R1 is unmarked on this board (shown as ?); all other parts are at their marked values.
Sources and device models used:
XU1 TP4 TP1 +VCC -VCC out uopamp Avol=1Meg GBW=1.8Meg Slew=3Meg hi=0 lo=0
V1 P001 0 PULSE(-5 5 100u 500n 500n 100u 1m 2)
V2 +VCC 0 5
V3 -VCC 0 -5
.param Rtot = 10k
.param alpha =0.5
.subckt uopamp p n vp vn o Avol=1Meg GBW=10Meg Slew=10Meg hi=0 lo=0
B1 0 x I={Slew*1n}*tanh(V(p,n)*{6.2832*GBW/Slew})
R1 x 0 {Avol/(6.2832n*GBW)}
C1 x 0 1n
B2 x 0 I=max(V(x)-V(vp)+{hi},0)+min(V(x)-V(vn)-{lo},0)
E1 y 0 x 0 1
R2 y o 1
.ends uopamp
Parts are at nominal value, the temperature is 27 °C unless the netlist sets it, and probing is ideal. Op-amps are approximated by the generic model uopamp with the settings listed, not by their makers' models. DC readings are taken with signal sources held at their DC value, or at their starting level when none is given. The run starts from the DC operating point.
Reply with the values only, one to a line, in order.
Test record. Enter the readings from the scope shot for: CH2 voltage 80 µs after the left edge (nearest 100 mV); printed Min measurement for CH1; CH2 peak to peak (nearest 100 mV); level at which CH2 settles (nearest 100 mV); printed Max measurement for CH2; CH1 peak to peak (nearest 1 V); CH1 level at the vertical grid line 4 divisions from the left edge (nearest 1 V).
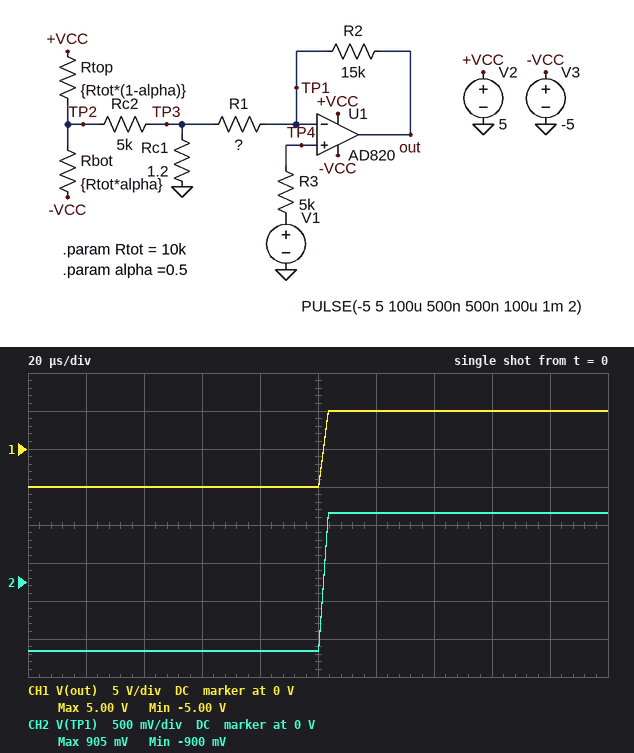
-900 mV
-5.00 V
1.8 V
900 mV
905 mV
10 V
-5 V
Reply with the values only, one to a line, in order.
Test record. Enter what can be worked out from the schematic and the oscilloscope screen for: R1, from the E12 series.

3.3 kΩ
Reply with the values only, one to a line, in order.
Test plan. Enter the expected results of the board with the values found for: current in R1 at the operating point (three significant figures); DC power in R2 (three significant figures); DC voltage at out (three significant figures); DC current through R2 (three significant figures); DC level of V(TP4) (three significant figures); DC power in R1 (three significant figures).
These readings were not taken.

273 µA
1.12 mW
-5.00 V
273 µA
-5.00 V
247 µW
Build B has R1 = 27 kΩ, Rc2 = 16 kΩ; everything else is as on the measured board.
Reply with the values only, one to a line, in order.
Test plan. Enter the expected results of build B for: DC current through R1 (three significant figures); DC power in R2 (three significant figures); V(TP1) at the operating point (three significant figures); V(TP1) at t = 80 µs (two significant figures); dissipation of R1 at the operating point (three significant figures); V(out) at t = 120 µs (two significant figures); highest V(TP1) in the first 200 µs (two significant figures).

119 µA
213 µW
-3.22 V
-3.2 V
383 µW
5.0 V
3.2 V
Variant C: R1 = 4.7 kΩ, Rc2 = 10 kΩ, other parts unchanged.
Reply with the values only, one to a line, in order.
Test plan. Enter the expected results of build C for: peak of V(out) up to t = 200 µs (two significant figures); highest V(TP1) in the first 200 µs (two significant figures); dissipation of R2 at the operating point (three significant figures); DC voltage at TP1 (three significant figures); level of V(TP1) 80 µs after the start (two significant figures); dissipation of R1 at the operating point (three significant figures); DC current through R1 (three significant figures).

5.0 V
1.2 V
967 µW
-1.19 V
-1.2 V
303 µW
254 µA
